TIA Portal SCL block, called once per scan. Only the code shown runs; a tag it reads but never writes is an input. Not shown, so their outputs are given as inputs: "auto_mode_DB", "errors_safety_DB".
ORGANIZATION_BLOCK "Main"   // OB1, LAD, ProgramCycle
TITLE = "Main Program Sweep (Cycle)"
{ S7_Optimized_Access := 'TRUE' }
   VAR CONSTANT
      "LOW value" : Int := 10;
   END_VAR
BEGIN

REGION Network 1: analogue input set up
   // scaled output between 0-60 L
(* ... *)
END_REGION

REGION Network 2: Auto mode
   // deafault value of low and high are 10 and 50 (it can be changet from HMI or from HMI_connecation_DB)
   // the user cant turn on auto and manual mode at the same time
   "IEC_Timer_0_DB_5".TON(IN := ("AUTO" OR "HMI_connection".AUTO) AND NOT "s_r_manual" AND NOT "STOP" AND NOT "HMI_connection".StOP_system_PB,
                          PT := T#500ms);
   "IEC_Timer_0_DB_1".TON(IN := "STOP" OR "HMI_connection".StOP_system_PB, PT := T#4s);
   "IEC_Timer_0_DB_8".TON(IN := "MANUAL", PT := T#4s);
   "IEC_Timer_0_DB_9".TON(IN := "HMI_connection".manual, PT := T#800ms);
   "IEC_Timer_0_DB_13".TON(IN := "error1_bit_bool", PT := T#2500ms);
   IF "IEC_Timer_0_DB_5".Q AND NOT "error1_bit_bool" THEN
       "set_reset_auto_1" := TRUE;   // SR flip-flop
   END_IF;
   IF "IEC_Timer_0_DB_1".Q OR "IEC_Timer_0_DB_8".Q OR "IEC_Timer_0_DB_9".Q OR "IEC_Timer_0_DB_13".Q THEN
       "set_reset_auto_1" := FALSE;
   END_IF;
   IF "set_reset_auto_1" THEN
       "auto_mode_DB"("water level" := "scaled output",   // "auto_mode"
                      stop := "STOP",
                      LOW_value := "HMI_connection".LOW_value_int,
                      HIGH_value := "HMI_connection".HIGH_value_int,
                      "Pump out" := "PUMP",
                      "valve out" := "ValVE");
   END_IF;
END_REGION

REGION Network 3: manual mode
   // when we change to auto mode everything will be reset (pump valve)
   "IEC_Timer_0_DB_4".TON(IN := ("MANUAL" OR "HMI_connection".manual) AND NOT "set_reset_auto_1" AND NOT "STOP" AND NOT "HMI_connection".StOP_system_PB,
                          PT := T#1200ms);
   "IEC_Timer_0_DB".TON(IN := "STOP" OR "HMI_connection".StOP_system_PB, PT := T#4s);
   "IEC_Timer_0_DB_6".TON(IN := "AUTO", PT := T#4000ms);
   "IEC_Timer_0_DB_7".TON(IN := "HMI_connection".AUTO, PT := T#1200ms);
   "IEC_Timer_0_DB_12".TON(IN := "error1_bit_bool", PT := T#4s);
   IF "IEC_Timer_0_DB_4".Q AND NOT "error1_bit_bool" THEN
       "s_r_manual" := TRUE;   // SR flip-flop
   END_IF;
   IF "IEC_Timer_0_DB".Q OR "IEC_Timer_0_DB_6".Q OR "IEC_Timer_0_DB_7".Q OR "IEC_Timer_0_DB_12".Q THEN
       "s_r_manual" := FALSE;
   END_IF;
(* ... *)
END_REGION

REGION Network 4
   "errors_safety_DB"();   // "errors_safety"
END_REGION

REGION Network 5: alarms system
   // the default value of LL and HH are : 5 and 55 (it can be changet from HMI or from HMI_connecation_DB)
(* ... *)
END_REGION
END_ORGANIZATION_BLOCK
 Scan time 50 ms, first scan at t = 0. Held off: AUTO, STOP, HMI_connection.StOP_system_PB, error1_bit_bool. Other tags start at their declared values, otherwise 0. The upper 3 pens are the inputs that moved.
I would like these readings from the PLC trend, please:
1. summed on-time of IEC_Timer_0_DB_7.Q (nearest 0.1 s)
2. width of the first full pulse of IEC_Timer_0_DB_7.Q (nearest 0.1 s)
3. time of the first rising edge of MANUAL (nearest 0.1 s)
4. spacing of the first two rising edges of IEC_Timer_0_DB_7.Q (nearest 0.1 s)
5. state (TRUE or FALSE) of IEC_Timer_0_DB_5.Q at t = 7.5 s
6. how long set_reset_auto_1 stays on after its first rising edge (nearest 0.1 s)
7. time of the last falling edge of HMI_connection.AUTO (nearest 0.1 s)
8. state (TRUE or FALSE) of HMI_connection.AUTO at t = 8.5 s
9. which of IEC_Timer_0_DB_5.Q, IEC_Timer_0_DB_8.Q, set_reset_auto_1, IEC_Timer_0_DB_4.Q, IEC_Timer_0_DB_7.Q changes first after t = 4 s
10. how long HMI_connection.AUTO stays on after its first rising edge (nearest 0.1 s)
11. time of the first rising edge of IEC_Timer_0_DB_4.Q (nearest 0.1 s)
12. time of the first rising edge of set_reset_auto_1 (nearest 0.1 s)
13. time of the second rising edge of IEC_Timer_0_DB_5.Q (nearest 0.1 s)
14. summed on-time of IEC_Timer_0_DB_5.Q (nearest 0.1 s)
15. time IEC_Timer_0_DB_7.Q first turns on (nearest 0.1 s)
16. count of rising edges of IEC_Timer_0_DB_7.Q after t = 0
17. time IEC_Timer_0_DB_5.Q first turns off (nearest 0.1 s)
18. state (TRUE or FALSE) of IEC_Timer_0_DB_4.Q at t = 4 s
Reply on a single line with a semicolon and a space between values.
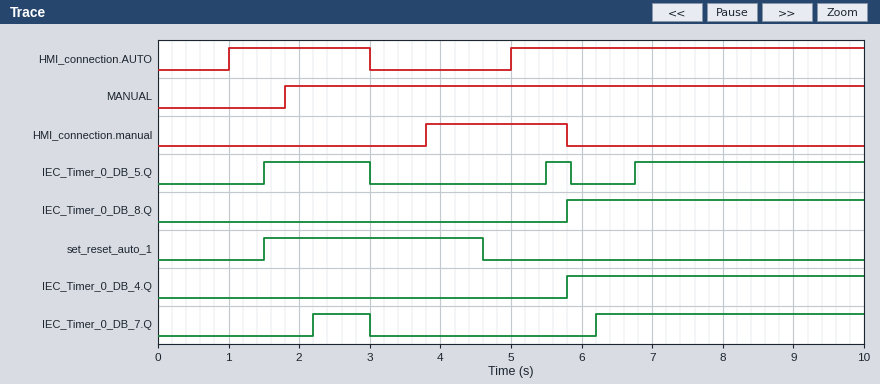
4.6 s; 0.8 s; 1.8 s; 4.0 s; TRUE; 3.1 s; 3.0 s; TRUE; set_reset_auto_1; 2.0 s; 5.8 s; 1.5 s; 5.5 s; 5.1 s; 2.2 s; 2; 3.0 s; FALSE
